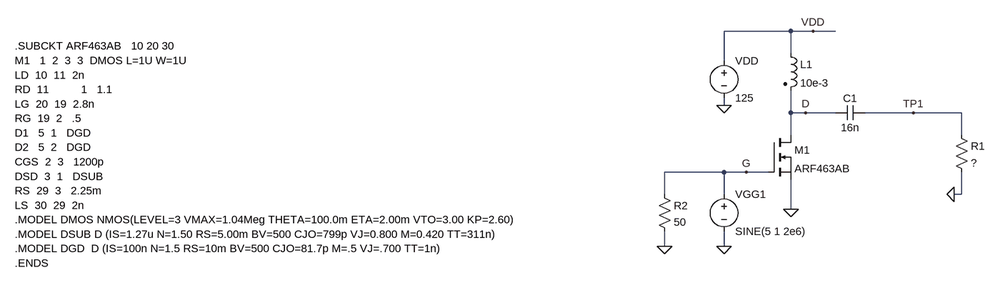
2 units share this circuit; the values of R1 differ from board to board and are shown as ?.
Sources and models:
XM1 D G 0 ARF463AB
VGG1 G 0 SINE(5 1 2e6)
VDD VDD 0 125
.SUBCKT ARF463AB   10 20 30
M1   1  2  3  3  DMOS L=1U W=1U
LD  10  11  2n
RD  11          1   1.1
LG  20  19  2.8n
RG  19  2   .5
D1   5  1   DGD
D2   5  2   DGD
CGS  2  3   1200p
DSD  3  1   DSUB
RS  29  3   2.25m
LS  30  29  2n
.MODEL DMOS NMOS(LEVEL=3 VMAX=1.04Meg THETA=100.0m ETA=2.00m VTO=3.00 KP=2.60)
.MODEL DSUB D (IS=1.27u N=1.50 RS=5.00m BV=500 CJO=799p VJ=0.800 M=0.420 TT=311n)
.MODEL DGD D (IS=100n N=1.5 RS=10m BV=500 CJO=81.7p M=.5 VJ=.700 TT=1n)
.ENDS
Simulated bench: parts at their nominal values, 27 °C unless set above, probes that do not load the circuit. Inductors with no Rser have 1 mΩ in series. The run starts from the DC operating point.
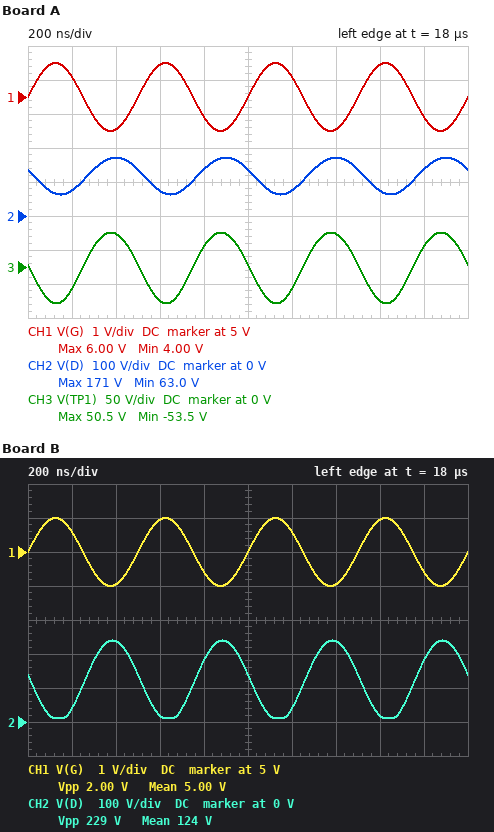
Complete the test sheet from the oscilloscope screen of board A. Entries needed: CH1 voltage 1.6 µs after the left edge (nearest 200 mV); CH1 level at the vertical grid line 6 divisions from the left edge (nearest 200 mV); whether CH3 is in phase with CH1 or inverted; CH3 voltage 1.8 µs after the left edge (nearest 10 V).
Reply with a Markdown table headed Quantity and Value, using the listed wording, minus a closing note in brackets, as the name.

| Quantity | Value |
|---|---|
| CH1 voltage 1.6 µs after the left edge | 6.0 V |
| CH1 level at the vertical grid line 6 divisions from the left edge | 5.6 V |
| whether CH3 is in phase with CH1 or inverted | inverted |
| CH3 voltage 1.8 µs after the left edge | 30 V |
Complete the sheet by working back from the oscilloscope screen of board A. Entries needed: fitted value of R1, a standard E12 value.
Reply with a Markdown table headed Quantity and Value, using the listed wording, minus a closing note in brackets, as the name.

| Quantity | Value |
|---|---|
| fitted value of R1, a standard E12 value | 18 Ω |
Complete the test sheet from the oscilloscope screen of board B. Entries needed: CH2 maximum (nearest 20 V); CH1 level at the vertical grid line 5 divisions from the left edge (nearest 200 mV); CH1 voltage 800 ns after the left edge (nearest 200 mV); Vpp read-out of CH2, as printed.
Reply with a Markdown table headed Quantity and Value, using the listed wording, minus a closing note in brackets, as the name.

| Quantity | Value |
|---|---|
| CH2 maximum | 240 V |
| CH1 level at the vertical grid line 5 divisions from the left edge | 5.0 V |
| CH1 voltage 800 ns after the left edge | 4.4 V |
| Vpp read-out of CH2, as printed | 229 V |
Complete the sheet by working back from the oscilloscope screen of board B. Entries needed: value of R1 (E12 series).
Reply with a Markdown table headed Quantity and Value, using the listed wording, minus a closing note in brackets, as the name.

| Quantity | Value |
|---|---|
| value of R1 | 68 Ω |
